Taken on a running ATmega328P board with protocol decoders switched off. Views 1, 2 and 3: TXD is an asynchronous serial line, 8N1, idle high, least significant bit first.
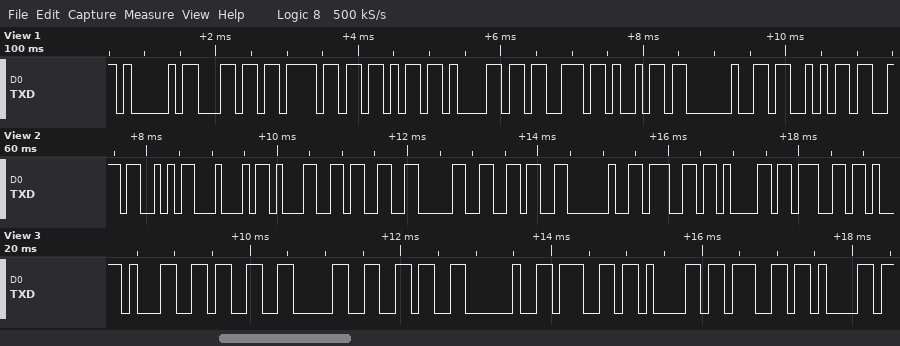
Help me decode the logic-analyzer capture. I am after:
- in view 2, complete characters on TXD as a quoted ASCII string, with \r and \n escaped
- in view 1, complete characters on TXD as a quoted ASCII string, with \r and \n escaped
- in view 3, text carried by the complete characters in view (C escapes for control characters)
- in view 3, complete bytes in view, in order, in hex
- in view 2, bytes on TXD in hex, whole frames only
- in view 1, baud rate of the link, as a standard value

"SD1306 gag"
"Alokasi S"
"1306 gaga"
31 33 30 36 20 67 61 67 61
53 44 31 33 30 36 20 67 61 67
9600 baud
